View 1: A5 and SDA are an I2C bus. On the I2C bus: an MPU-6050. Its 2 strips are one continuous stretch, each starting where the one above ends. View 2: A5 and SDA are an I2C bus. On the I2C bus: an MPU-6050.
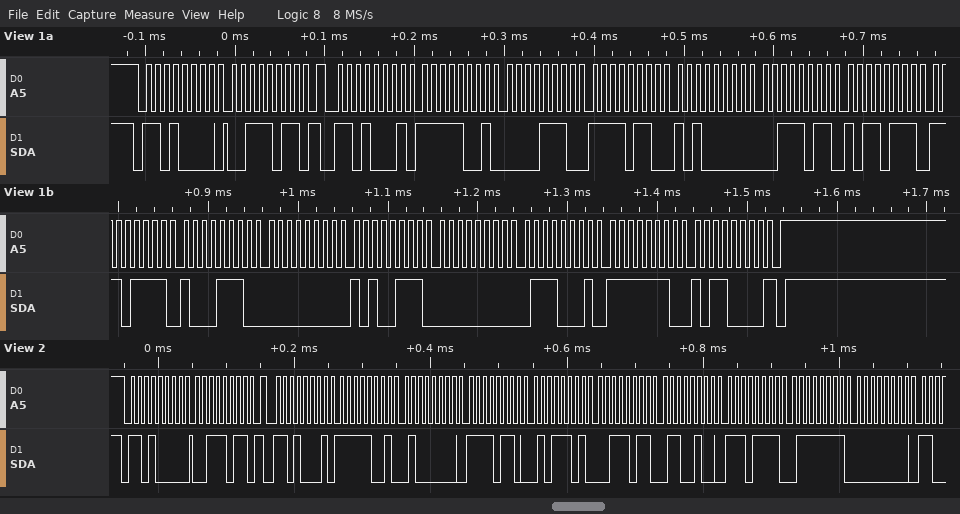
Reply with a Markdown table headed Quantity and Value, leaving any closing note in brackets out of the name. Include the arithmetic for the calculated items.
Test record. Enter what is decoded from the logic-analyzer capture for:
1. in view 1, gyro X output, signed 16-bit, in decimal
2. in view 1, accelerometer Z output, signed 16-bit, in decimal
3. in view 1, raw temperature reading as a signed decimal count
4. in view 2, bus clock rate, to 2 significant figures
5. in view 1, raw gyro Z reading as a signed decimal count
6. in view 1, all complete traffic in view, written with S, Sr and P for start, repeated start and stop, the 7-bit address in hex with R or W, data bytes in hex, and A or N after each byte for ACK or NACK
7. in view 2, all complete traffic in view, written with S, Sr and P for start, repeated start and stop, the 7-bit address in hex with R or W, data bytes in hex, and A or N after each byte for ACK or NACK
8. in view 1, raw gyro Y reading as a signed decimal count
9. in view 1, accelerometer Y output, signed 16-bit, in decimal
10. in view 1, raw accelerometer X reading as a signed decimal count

| Quantity | Value |
|---|---|
| in view 1, gyro X output, signed 16-bit, in decimal | 0x00A7 = 167 |
| in view 1, accelerometer Z output, signed 16-bit, in decimal | 0x3BB7 = 15287 |
| in view 1, raw temperature reading as a signed decimal count | 0xEF8E = -4210 |
| in view 2, bus clock rate, to 2 significant figures | 100 kHz |
| in view 1, raw gyro Z reading as a signed decimal count | 0xFEB0 = -336 |
| in view 1, all complete traffic in view, written with S, Sr and P for start, repeated start and stop, the 7-bit address in hex with R or W, data bytes in hex, and A or N after each byte for ACK or NACK | S 68W A 3B A Sr 68R A F9 A 0E A F6 A A0 A 3B A B7 A EF A 8E A 00 A A7 A 00 A 71 A FE A B0 N P |
| in view 2, all complete traffic in view, written with S, Sr and P for start, repeated start and stop, the 7-bit address in hex with R or W, data bytes in hex, and A or N after each byte for ACK or NACK | S 68W A 3B A Sr 68R A F9 A 40 A F6 A 5D A 3B A 64 A EF A 7F A 00 A |
| in view 1, raw gyro Y reading as a signed decimal count | 0x0071 = 113 |
| in view 1, accelerometer Y output, signed 16-bit, in decimal | 0xF6A0 = -2400 |
| in view 1, raw accelerometer X reading as a signed decimal count | 0xF90E = -1778 |
